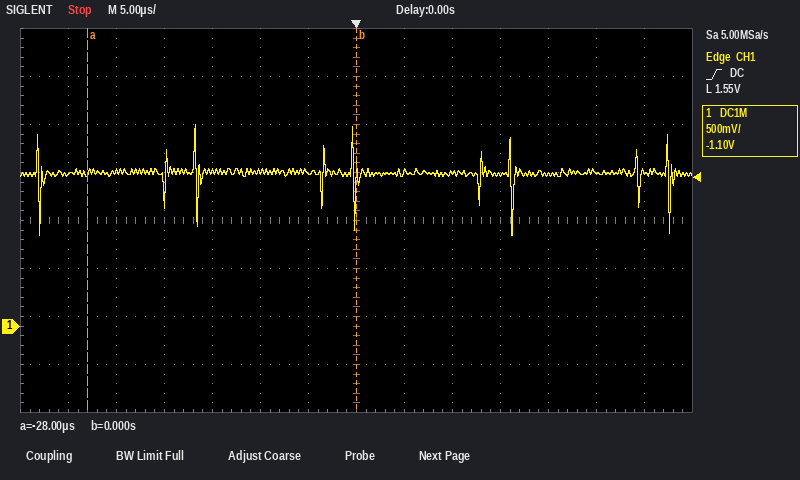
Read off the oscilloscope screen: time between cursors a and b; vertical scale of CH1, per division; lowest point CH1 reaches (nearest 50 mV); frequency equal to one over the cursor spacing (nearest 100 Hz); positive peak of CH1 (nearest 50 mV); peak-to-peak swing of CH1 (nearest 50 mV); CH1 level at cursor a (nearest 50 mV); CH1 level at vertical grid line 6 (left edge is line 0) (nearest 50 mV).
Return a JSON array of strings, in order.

["28.0 µs", "500 mV", "950 mV", "35.7 kHz", "2.10 V", "1.15 V", "1.60 V", "1.60 V"]
